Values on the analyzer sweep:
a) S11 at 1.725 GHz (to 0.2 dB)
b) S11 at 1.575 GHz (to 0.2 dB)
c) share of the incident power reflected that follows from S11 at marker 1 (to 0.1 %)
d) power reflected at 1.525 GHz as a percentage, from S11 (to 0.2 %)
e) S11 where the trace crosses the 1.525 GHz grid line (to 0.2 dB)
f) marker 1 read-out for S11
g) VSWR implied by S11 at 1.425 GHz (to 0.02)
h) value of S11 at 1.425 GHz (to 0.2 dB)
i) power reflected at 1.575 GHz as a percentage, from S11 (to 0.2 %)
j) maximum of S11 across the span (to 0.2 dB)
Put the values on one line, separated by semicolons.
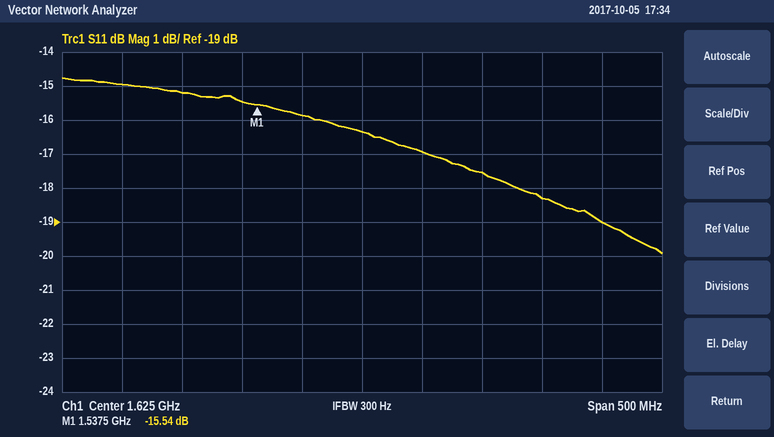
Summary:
-17.6 dB; -15.8 dB; 2.8 %; 2.8 %; -15.4 dB; -15.54 dB; 1.44; -15.0 dB; 2.6 %; -14.8 dB
